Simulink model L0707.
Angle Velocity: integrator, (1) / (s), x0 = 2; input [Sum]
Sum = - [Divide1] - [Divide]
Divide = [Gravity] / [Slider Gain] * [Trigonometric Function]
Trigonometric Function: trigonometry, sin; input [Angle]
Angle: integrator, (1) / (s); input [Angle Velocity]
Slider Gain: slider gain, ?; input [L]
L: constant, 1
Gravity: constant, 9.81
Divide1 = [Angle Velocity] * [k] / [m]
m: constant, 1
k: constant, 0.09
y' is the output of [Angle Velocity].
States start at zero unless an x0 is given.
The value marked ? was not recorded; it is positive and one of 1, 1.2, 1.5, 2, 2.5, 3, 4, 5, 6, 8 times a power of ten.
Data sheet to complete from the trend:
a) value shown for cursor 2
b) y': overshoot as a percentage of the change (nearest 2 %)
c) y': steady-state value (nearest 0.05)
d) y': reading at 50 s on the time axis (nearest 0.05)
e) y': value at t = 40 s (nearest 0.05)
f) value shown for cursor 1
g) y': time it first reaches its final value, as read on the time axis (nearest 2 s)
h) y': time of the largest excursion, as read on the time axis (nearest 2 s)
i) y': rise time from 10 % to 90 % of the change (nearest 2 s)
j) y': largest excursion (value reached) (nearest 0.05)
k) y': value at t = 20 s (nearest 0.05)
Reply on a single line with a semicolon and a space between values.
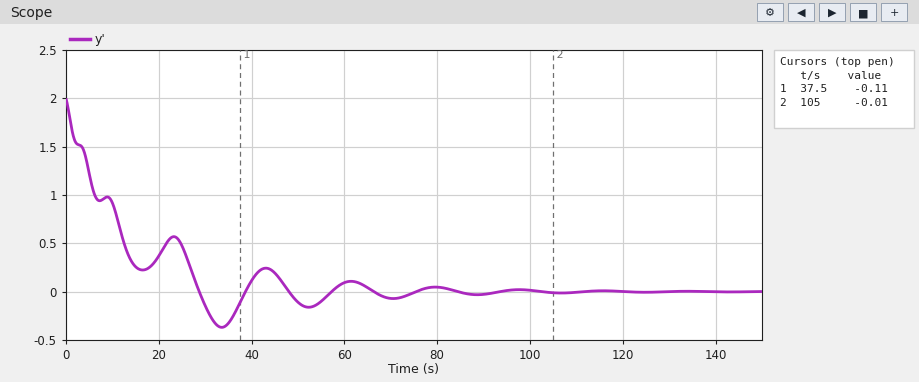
-0.01; 18 %; 0.00; -0.10; 0.10; -0.11; 28 s; 34 s; 26 s; -0.35; 0.35
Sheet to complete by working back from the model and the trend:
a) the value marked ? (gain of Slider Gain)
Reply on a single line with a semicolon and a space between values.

80
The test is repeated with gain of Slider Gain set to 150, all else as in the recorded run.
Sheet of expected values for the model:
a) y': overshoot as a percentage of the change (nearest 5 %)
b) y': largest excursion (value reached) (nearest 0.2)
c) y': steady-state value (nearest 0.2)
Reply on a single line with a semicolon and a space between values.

15 %; -0.2; 0.0
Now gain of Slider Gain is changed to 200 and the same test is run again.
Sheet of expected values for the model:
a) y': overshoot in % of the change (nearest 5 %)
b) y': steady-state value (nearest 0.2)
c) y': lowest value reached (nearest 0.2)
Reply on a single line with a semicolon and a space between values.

10 %; 0.0; -0.2
